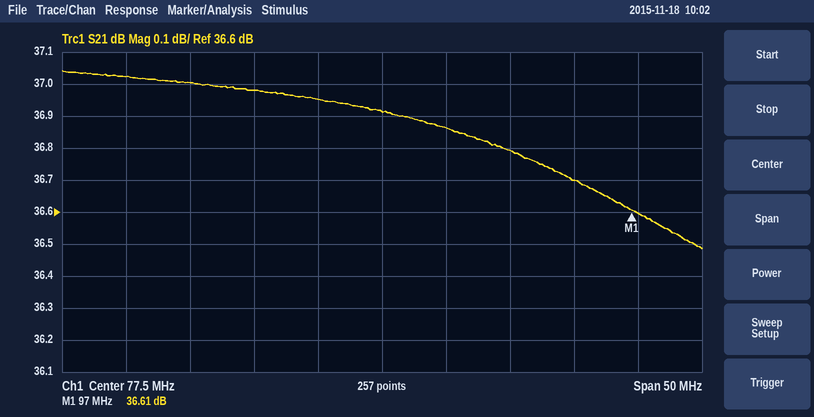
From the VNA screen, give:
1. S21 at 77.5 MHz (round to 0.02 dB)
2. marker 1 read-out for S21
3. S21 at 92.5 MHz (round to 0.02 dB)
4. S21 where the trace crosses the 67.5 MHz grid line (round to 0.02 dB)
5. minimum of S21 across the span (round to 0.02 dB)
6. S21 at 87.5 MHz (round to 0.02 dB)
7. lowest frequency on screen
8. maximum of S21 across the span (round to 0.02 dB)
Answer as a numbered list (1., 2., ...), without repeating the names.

1. 36.92 dB
2. 36.61 dB
3. 36.70 dB
4. 36.98 dB
5. 36.48 dB
6. 36.80 dB
7. 52.5 MHz
8. 37.04 dB
